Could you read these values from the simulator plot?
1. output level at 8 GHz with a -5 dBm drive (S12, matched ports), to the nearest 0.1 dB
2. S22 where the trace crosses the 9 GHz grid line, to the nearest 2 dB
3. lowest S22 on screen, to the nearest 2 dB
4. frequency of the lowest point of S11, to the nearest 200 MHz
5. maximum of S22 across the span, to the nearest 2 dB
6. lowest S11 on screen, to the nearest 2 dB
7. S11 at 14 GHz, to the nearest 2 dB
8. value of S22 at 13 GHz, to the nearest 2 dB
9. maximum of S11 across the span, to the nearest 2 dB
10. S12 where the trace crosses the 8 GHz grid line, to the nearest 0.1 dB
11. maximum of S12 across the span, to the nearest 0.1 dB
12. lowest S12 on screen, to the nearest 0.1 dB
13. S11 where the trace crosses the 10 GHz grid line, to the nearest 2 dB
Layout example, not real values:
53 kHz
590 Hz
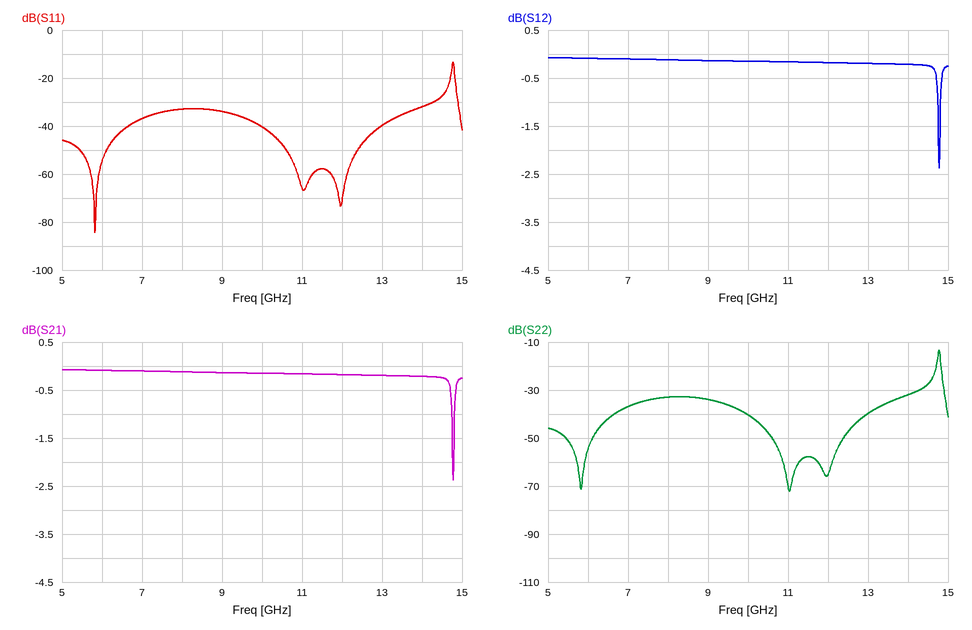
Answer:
-5.1 dBm
-34 dB
-72 dB
5.8 GHz
-14 dB
-84 dB
-32 dB
-40 dB
-14 dB
-0.1 dB
-0.1 dB
-2.4 dB
-40 dB
